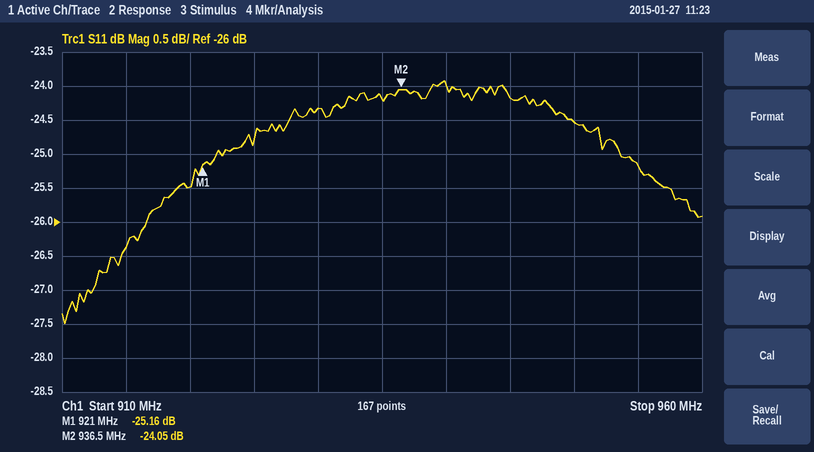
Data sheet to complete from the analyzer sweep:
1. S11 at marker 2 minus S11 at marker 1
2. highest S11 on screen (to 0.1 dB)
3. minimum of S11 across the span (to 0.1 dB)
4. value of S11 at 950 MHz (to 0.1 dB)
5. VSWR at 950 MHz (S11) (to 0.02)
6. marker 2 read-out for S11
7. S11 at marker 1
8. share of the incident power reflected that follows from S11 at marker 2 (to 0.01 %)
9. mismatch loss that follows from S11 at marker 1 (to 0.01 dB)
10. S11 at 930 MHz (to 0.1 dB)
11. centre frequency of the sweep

1.11 dB
-23.9 dB
-27.5 dB
-24.5 dB
1.12
-24.05 dB
-25.16 dB
0.39 %
0.01 dB
-24.3 dB
935 MHz
